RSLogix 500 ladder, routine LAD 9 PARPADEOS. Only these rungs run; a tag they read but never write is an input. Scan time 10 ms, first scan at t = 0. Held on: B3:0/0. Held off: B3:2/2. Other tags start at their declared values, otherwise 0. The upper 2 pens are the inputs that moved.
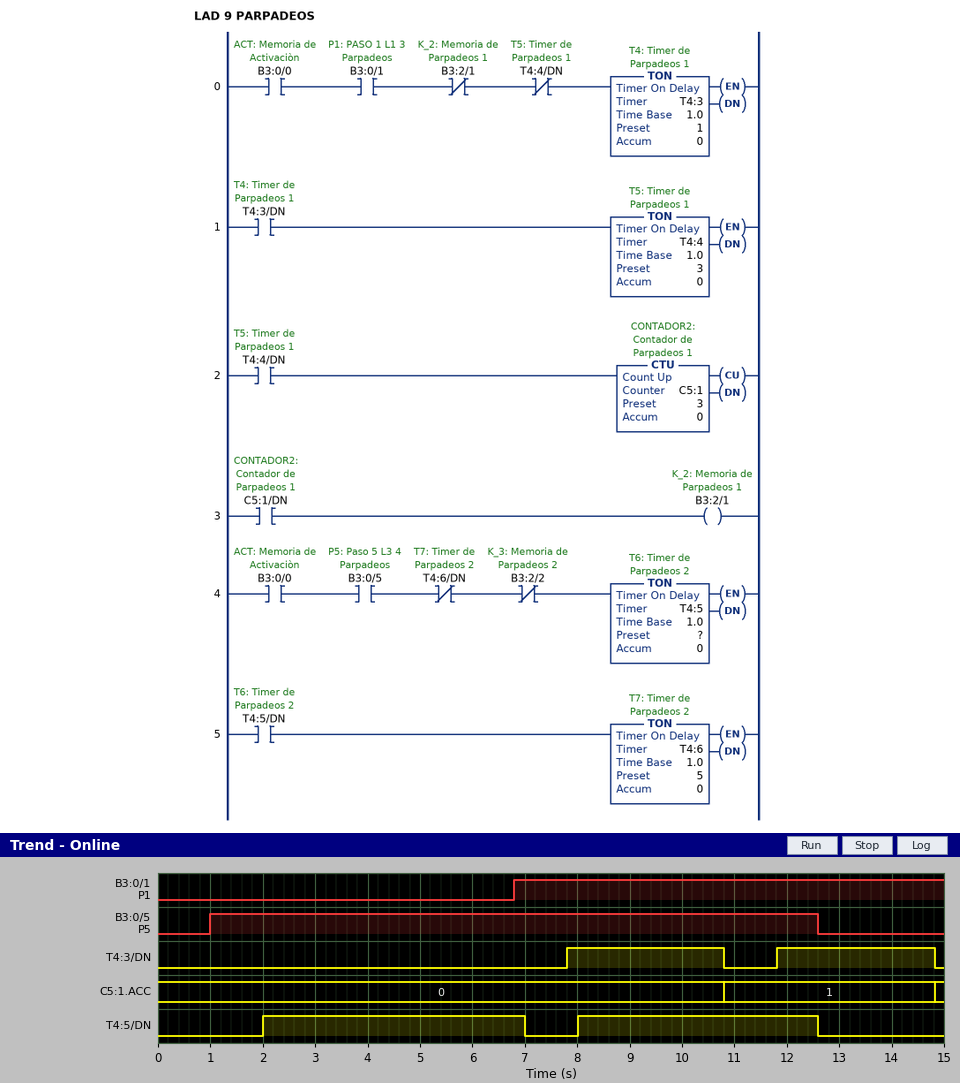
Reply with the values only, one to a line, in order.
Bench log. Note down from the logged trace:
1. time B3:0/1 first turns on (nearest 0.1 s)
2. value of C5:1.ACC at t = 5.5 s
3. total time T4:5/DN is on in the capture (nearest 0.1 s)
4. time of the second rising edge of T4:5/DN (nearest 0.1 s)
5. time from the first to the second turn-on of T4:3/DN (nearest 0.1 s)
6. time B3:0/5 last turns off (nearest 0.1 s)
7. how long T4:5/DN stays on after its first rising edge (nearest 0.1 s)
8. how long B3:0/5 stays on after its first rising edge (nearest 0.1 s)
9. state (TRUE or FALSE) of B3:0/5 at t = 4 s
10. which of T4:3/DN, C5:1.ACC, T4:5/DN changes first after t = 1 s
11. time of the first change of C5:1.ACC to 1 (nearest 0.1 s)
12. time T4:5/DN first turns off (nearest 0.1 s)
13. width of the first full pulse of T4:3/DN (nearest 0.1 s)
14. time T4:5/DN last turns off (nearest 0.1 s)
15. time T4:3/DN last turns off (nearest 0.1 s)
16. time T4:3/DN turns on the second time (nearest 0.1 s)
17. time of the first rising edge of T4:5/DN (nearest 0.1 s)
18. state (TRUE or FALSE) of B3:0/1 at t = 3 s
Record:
6.8 s
0
9.6 s
8.0 s
4.0 s
12.6 s
5.0 s
11.6 s
TRUE
T4:5/DN
10.8 s
7.0 s
3.0 s
12.6 s
14.8 s
11.8 s
2.0 s
FALSE
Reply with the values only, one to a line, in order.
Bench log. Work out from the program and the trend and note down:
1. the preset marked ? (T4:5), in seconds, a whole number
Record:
1 s
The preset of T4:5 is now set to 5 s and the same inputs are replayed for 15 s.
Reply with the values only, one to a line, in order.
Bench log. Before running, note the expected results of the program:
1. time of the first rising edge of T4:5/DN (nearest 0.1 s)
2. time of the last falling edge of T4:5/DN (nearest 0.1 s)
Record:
6.0 s
11.0 s
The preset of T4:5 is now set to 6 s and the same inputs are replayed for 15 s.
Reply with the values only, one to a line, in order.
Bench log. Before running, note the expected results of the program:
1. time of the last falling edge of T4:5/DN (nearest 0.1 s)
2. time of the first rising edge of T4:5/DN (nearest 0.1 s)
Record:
12.0 s
7.0 s
